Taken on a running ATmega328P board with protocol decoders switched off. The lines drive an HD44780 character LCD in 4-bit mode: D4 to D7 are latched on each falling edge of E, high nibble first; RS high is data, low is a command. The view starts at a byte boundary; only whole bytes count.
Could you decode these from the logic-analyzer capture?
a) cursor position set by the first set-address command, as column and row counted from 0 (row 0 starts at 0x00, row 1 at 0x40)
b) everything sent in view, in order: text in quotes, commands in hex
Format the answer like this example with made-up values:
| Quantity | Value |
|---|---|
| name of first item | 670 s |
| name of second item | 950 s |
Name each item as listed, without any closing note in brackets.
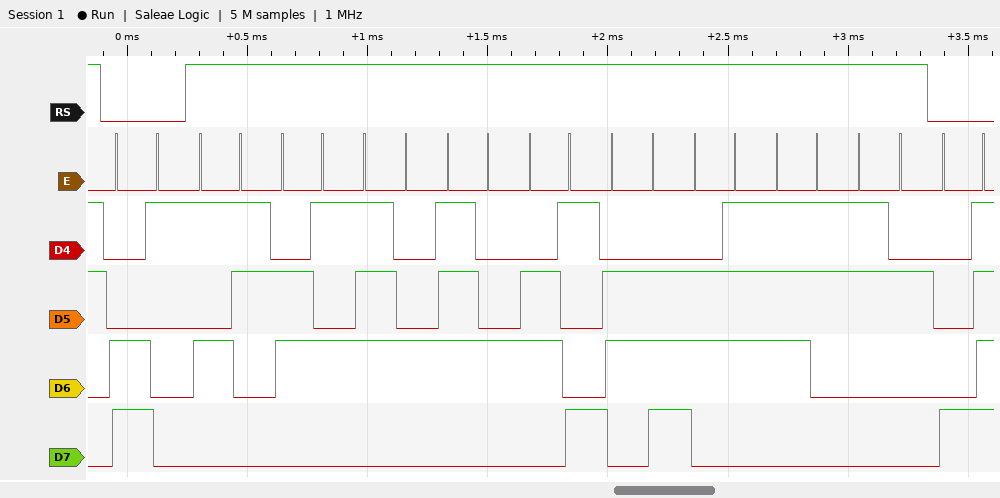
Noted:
| Quantity | Value |
|---|---|
| cursor position set by the first set-address command, as column and row counted from 0 | column 1, row 1 |
| everything sent in view, in order: text in quotes, commands in hex | 0xC1 "Settings2" 0x8F |
